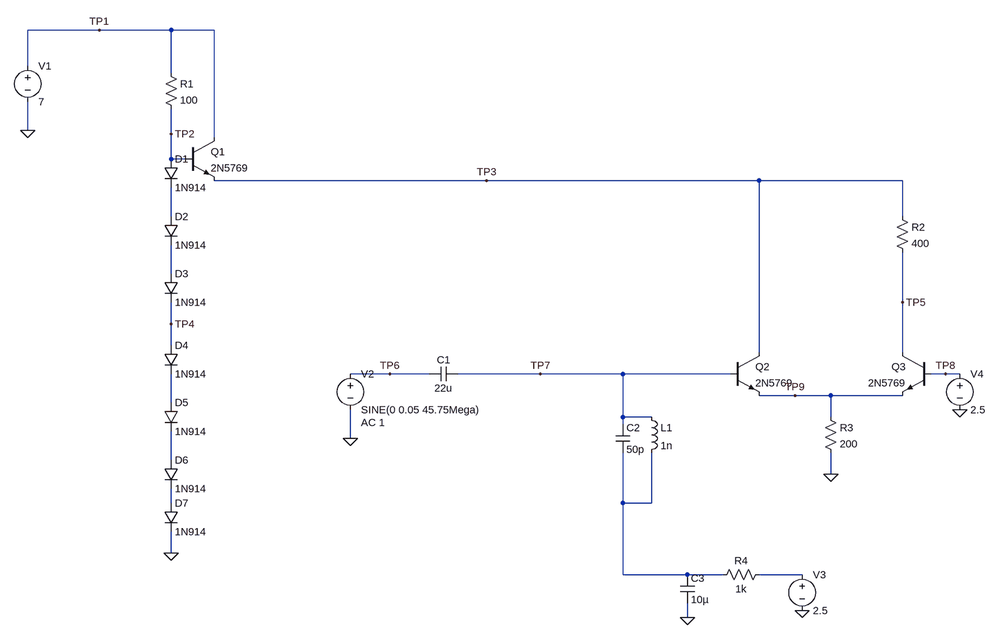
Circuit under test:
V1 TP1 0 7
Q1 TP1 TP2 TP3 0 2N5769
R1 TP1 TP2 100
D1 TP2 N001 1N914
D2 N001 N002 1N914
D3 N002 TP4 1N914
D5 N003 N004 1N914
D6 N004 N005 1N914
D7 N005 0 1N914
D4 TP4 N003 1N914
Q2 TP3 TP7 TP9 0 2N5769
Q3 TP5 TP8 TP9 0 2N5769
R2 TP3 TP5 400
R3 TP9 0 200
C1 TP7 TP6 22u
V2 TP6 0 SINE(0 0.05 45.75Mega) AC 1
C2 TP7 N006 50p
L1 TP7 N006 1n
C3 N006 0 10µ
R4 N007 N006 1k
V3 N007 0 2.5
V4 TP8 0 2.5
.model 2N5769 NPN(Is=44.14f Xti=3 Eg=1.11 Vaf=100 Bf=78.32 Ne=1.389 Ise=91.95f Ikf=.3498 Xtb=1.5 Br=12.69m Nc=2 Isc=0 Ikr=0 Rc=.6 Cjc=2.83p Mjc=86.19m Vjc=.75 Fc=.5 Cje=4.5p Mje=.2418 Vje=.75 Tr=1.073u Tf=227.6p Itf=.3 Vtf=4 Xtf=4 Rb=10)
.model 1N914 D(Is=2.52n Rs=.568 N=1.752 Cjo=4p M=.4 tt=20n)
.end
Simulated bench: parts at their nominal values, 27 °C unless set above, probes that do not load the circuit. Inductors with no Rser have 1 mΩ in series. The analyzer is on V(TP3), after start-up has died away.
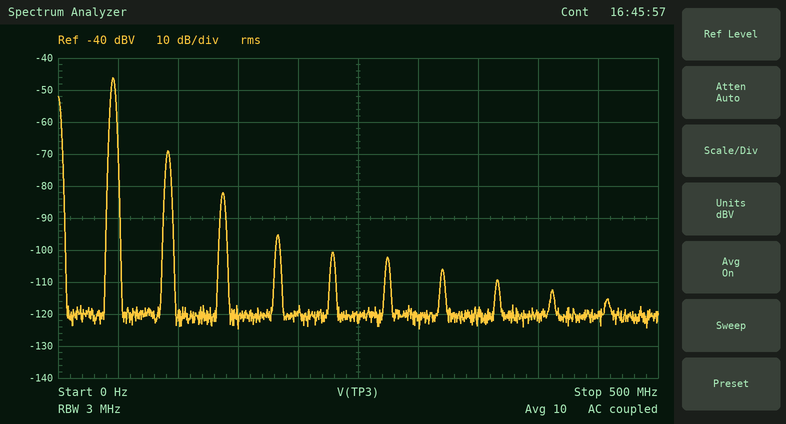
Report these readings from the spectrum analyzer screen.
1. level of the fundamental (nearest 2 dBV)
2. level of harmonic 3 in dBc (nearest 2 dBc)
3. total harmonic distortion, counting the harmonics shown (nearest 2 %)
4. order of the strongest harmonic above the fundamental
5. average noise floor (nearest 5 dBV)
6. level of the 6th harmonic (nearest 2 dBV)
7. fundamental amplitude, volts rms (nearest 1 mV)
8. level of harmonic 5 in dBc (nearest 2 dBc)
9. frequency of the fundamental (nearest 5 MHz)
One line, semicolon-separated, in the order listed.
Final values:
-46 dBV; -36 dBc; 8 %; 2; -120 dBV; -102 dBV; 5 mV; -54 dBc; 45 MHz
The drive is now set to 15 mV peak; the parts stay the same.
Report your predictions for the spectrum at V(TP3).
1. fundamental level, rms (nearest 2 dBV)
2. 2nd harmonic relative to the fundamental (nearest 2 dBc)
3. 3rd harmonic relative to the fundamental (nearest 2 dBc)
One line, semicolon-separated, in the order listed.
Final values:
-56 dBV; -34 dBc; -54 dBc
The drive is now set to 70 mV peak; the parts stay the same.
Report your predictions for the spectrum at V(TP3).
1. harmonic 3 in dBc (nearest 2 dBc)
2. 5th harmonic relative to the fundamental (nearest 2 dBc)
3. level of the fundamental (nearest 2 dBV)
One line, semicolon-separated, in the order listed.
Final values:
-28 dBc; -30 dBc; -44 dBV
